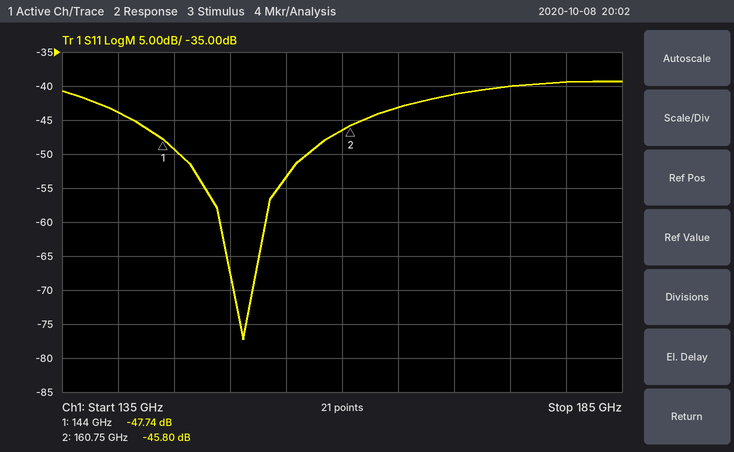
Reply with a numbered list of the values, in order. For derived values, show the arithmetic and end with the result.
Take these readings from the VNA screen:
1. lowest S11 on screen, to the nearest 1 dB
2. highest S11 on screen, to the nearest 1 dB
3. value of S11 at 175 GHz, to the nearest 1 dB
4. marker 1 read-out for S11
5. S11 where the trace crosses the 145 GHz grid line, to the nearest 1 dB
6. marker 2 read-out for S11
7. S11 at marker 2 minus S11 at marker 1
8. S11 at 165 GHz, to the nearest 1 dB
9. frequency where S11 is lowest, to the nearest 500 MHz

1. -77 dB
2. -39 dB
3. -40 dB
4. -47.74 dB
5. -49 dB
6. -45.80 dB
7. -45.8 − (-47.74) = 1.94 dB
8. -43 dB
9. 151.0 GHz
